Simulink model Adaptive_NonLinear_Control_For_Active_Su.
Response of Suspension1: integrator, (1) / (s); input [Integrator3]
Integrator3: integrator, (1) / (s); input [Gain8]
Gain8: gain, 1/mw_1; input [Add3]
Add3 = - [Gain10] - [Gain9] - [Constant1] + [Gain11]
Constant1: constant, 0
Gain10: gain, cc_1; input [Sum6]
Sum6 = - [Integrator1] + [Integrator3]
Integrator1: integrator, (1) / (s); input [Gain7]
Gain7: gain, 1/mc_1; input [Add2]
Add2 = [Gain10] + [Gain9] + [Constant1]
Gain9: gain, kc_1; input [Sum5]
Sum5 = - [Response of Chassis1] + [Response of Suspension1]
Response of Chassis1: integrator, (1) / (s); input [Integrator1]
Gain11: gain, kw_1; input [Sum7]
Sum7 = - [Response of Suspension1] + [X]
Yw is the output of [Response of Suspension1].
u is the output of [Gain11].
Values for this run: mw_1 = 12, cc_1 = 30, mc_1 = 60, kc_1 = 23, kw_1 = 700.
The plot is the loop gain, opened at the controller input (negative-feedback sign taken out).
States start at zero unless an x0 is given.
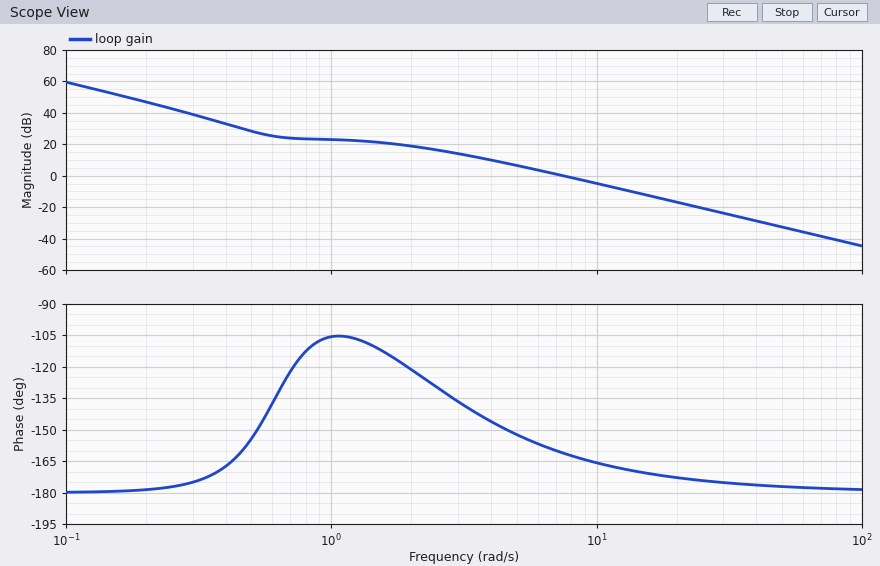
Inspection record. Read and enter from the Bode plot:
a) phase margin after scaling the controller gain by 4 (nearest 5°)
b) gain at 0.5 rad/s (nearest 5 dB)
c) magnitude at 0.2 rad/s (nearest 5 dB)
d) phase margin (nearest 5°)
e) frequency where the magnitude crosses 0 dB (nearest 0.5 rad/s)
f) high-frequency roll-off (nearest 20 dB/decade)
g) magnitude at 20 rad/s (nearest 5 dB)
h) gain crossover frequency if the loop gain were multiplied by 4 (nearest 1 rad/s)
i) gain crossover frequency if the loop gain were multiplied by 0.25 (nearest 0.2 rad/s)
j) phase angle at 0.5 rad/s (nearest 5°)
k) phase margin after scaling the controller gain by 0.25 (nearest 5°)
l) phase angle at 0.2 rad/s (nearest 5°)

10°
30 dB
45 dB
20°
7.5 rad/s
-40 dB/decade
-15 dB
15 rad/s
3.4 rad/s
-155°
40°
-180°
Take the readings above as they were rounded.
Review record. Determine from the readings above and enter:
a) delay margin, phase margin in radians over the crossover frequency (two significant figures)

0.047 s
